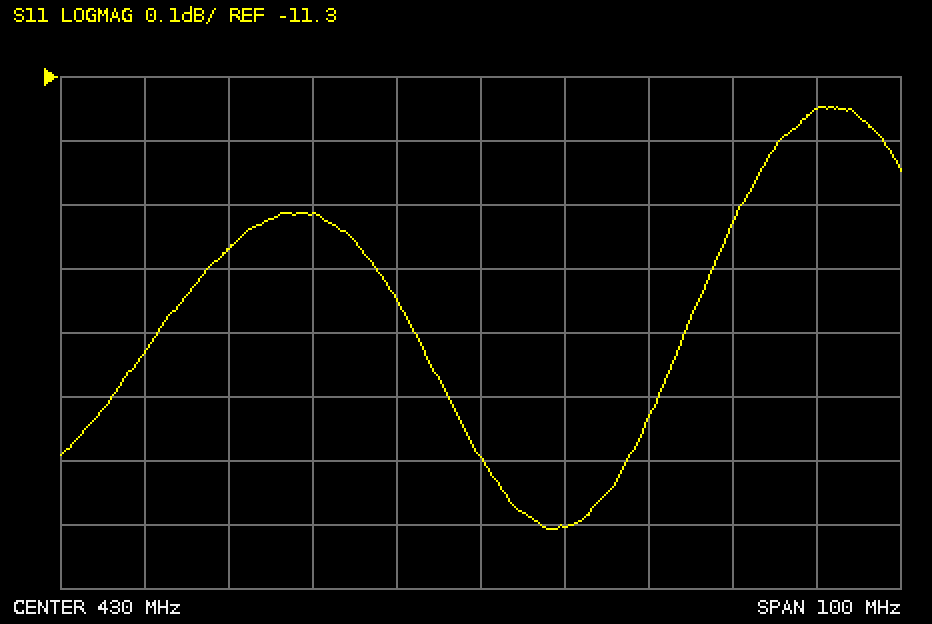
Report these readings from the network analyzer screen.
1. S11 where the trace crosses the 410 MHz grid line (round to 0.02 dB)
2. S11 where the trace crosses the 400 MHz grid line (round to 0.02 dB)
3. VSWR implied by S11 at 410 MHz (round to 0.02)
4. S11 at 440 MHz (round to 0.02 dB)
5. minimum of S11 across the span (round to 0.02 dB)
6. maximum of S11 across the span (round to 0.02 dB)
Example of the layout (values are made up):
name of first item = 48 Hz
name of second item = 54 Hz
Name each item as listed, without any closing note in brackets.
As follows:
S11 where the trace crosses the 410 MHz grid line = -11.52 dB
S11 where the trace crosses the 400 MHz grid line = -11.56 dB
VSWR implied by S11 at 410 MHz = 1.72
S11 at 440 MHz = -12.00 dB
minimum of S11 across the span = -12.00 dB
maximum of S11 across the span = -11.34 dB
